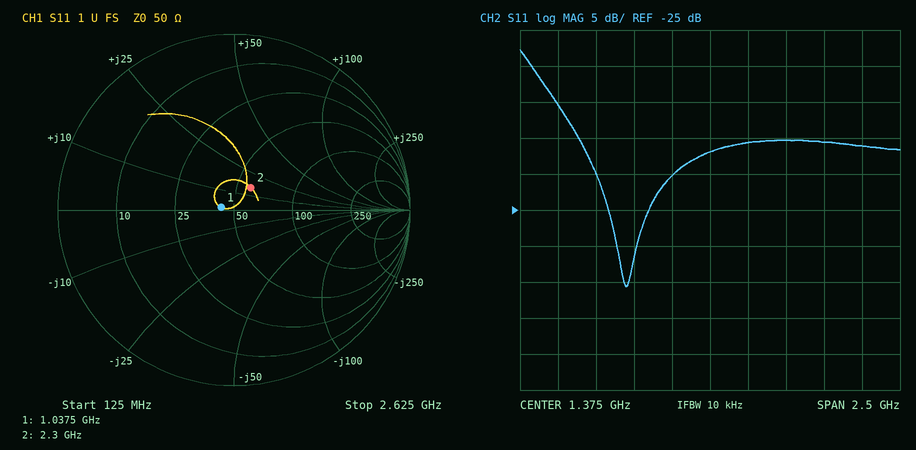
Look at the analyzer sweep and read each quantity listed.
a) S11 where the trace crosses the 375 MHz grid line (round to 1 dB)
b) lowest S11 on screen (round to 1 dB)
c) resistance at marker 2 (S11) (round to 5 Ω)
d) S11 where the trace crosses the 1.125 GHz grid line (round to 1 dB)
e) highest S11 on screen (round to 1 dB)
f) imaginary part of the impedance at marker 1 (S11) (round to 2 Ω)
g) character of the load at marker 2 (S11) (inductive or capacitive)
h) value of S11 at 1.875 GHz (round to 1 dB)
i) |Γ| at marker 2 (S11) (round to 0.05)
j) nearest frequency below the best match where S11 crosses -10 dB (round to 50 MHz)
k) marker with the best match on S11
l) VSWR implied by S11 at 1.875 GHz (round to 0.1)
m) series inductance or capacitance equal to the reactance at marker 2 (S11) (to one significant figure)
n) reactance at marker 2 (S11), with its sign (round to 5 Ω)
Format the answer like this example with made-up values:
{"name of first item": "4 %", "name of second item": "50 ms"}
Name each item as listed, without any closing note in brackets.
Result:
{"S11 where the trace crosses the 375 MHz grid line": "-10 dB", "lowest S11 on screen": "-36 dB", "resistance at marker 2 (S11)": "60 Ω", "S11 where the trace crosses the 1.125 GHz grid line": "-20 dB", "highest S11 on screen": "-3 dB", "imaginary part of the impedance at marker 1 (S11)": "+2 Ω", "character of the load at marker 2 (S11)": "inductive", "value of S11 at 1.875 GHz": "-15 dB", "|Γ| at marker 2 (S11)": "0.15", "nearest frequency below the best match where S11 crosses -10 dB": "350 MHz", "marker with the best match on S11": "marker 1", "VSWR implied by S11 at 1.875 GHz": "1.4", "series inductance or capacitance equal to the reactance at marker 2 (S11)": "1 nH", "reactance at marker 2 (S11), with its sign": "+15 Ω"}
